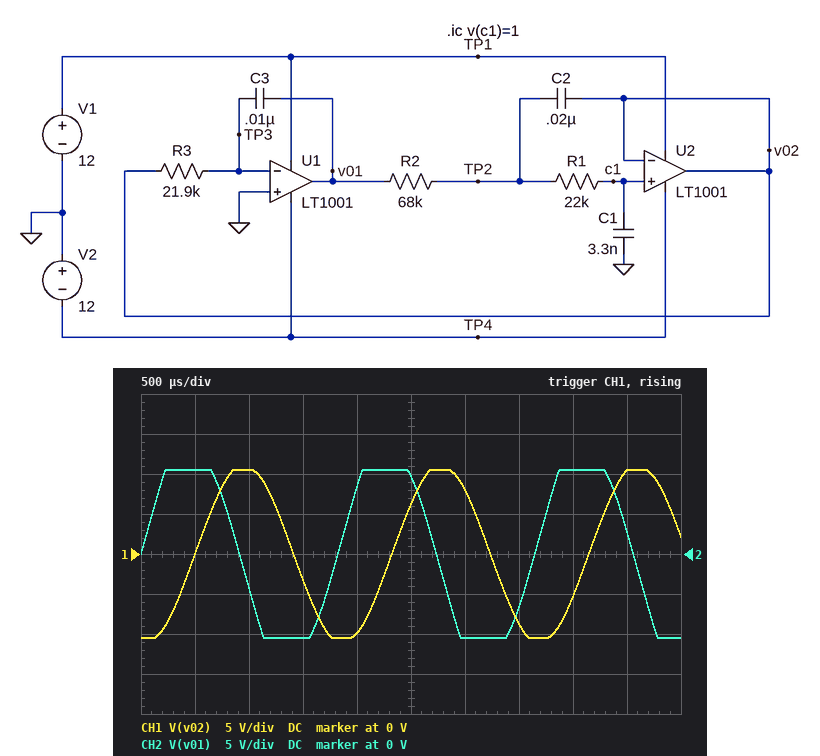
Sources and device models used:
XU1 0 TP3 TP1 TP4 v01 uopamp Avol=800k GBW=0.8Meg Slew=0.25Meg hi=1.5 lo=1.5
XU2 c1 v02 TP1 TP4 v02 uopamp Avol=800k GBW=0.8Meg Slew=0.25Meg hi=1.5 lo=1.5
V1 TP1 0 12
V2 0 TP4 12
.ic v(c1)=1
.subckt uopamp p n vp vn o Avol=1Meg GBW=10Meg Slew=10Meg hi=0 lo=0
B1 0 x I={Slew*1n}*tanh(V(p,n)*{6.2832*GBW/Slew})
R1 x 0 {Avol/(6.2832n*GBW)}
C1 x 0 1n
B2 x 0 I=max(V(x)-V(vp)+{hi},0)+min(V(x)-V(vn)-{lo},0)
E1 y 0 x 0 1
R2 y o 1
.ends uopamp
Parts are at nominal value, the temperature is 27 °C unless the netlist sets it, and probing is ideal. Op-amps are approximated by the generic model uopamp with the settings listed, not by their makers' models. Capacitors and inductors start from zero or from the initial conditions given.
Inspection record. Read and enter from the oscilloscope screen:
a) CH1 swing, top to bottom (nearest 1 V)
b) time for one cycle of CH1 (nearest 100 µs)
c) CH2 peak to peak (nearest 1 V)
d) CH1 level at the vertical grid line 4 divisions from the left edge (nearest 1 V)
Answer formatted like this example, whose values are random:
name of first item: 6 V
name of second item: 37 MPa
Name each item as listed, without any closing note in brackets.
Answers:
CH1 swing, top to bottom: 21 V
time for one cycle of CH1: 1.8 ms
CH2 peak to peak: 21 V
CH1 level at the vertical grid line 4 divisions from the left edge: -10 V
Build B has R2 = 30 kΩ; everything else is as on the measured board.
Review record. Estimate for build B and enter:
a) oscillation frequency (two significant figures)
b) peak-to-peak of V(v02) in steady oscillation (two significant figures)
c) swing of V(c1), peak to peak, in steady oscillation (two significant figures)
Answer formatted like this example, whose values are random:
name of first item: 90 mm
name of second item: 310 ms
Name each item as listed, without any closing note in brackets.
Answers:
oscillation frequency: 760 Hz
peak-to-peak of V(v02) in steady oscillation: 21 V
swing of V(c1), peak to peak, in steady oscillation: 23 V
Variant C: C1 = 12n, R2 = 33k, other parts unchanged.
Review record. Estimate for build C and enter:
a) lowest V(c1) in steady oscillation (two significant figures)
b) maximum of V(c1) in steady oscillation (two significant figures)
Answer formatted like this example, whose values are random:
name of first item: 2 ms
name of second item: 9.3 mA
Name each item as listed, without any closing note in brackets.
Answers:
lowest V(c1) in steady oscillation: -6.8 V
maximum of V(c1) in steady oscillation: 6.8 V
